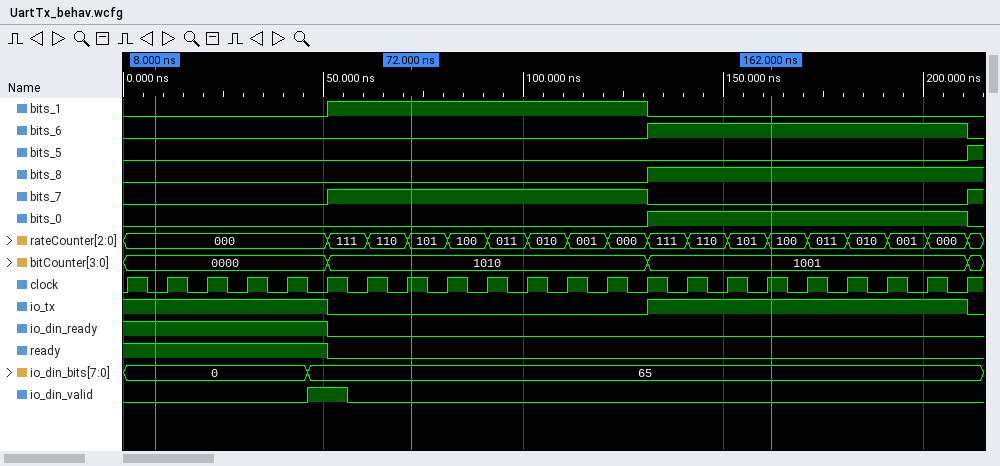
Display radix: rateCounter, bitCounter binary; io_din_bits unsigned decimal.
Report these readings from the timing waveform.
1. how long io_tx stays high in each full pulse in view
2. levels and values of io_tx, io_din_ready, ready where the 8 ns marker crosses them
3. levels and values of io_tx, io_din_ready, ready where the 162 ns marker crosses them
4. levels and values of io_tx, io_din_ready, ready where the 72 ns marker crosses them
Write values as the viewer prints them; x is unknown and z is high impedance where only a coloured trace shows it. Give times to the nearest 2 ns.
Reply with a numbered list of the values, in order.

1. 80 ns
2. io_tx=1, io_din_ready=1, ready=1
3. io_tx=1, io_din_ready=0, ready=0
4. io_tx=0, io_din_ready=0, ready=0
